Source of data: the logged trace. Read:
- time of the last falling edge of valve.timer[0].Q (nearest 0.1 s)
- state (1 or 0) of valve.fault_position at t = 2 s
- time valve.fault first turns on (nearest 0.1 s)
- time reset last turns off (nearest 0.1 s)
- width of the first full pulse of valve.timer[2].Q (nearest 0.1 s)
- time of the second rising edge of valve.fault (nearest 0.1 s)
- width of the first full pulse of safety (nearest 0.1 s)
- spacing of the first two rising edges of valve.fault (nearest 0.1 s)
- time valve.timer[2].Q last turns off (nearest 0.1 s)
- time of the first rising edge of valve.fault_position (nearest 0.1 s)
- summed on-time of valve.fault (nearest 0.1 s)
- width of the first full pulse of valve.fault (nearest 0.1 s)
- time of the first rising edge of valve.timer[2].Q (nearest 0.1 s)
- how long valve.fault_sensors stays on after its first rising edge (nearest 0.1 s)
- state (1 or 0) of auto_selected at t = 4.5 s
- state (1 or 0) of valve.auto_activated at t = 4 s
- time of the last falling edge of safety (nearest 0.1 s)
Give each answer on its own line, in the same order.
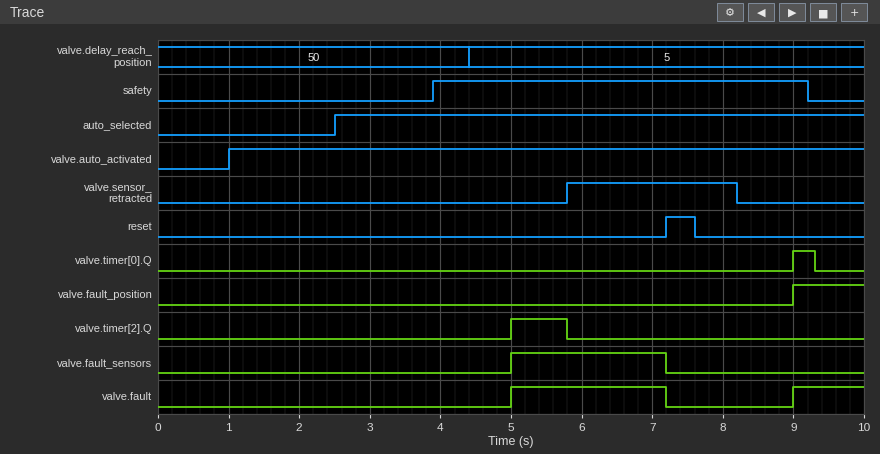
9.3 s
0
5.0 s
7.6 s
0.8 s
9.0 s
5.3 s
4.0 s
5.8 s
9.0 s
3.2 s
2.2 s
5.0 s
2.2 s
1
1
9.2 s
